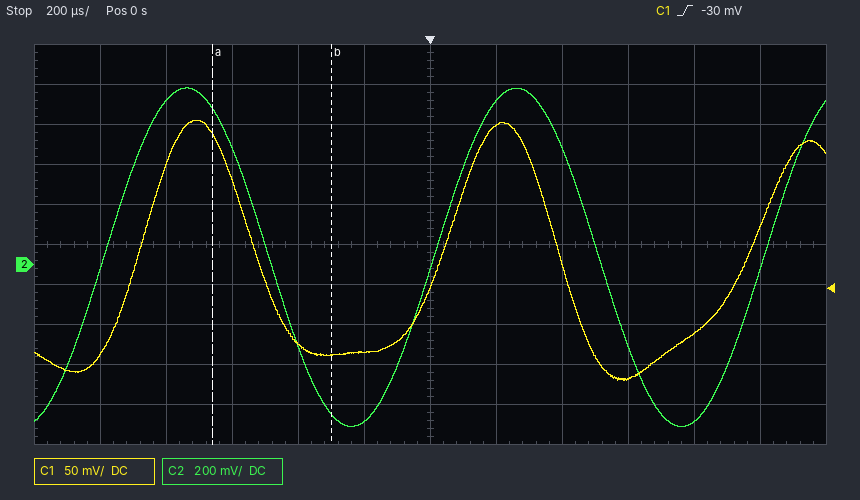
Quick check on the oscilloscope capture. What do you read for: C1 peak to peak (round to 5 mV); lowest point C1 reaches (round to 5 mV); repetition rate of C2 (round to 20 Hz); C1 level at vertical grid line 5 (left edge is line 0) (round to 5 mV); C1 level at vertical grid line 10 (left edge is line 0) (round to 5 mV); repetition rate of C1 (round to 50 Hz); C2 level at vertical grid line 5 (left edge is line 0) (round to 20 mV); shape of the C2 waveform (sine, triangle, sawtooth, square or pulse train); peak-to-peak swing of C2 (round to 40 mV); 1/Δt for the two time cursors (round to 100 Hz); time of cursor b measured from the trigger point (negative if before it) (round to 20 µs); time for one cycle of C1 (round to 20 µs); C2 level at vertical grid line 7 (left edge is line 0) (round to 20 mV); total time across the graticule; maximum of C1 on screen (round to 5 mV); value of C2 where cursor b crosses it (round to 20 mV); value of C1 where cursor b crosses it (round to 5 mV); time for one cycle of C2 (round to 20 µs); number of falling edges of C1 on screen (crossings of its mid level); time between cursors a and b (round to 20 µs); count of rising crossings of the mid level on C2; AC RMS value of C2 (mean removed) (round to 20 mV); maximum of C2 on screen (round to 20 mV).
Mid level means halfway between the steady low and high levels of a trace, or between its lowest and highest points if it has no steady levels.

325 mV
-145 mV
1.00 kHz
-110 mV
-85 mV
1.10 kHz
-780 mV
sine
1.68 V
2.8 kHz
-300 µs
920 µs
820 mV
2.4 ms
180 mV
-740 mV
-115 mV
1.00 ms
2
360 µs
3
600 mV
880 mV
